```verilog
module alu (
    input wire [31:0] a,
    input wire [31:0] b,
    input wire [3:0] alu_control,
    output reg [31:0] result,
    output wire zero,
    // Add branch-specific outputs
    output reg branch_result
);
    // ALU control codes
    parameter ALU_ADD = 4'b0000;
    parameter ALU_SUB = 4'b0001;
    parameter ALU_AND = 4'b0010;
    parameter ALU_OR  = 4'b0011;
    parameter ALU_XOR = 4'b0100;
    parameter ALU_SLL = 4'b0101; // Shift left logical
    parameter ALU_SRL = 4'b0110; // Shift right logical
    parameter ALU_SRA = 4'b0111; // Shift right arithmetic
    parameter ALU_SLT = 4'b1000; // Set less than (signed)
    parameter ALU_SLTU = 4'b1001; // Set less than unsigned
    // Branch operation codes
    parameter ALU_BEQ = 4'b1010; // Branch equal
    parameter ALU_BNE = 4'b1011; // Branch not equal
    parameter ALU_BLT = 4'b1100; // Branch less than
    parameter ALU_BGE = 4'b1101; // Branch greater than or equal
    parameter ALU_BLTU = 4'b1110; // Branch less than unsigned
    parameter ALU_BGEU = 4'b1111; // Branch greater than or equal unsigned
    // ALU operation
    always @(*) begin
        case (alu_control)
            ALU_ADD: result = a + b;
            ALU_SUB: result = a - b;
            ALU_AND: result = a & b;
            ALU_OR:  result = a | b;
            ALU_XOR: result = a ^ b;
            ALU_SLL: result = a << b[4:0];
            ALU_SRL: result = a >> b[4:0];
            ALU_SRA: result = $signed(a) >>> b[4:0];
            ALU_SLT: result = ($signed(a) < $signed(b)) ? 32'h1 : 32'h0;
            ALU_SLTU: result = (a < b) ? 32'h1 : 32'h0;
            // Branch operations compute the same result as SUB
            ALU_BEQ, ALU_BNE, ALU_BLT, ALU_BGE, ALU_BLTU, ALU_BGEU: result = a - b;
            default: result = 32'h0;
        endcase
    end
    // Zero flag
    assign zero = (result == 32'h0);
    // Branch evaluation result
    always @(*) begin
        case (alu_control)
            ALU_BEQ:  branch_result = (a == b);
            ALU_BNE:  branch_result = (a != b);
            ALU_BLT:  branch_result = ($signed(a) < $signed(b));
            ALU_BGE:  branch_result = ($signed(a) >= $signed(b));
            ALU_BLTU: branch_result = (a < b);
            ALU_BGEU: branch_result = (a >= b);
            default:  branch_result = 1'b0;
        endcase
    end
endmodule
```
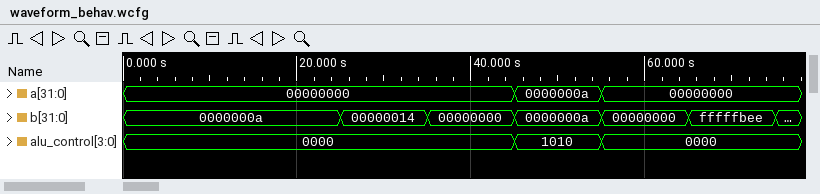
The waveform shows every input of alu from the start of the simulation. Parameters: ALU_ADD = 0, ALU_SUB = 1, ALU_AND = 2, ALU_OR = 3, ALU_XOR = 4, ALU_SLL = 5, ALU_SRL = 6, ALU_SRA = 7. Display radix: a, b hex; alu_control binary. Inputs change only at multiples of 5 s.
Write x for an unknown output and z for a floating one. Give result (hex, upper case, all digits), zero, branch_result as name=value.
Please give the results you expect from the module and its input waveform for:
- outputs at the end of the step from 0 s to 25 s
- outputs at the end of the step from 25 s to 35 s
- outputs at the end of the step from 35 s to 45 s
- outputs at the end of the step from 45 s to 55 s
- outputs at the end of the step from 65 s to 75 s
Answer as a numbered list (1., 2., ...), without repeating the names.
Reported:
1. result=0000000A, zero=0, branch_result=0
2. result=00000014, zero=0, branch_result=0
3. result=00000000, zero=1, branch_result=0
4. result=00000000, zero=1, branch_result=1
5. result=FFFFFBEE, zero=0, branch_result=0
